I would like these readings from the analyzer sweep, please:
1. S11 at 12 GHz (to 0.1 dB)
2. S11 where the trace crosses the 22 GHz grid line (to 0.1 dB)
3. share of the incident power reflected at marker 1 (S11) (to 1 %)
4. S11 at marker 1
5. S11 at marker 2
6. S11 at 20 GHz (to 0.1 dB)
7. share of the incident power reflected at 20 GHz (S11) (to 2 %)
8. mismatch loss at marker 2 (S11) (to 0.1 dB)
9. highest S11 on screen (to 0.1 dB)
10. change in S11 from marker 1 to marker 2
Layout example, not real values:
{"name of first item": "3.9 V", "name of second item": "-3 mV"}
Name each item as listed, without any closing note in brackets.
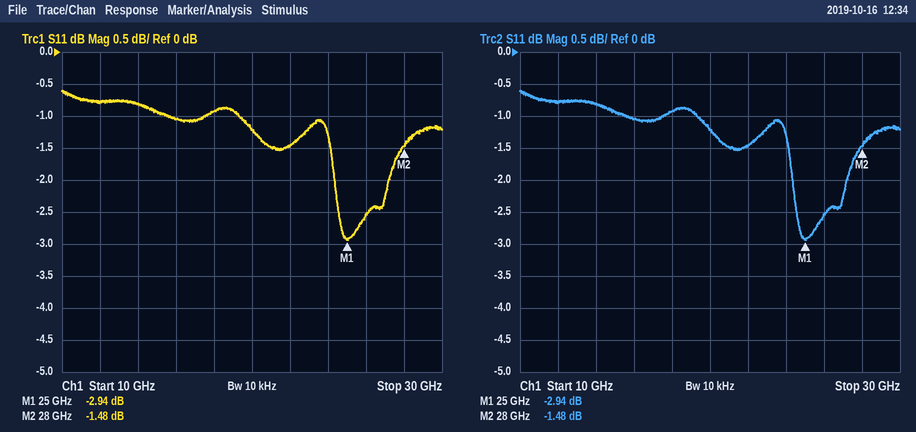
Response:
{"S11 at 12 GHz": "-0.8 dB", "S11 where the trace crosses the 22 GHz grid line": "-1.5 dB", "share of the incident power reflected at marker 1 (S11)": "51 %", "S11 at marker 1": "-2.94 dB", "S11 at marker 2": "-1.48 dB", "S11 at 20 GHz": "-1.2 dB", "share of the incident power reflected at 20 GHz (S11)": "76 %", "mismatch loss at marker 2 (S11)": "5.4 dB", "highest S11 on screen": "-0.6 dB", "change in S11 from marker 1 to marker 2": "1.46 dB"}
